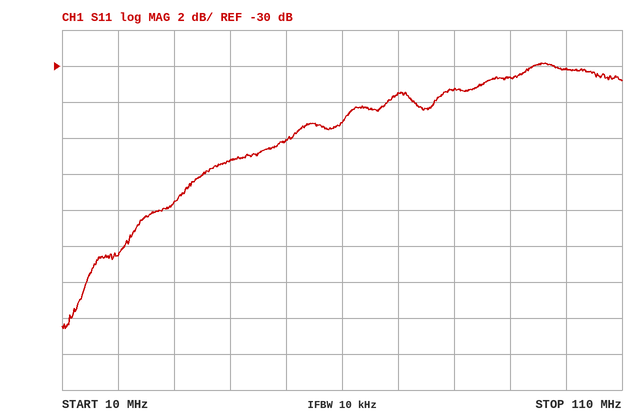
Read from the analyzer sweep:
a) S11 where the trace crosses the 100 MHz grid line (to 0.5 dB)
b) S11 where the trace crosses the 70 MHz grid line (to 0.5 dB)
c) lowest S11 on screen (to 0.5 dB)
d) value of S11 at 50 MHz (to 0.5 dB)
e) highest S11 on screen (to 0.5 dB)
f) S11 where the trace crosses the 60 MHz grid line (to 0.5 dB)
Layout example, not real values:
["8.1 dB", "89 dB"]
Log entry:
["-30.0 dB", "-31.5 dB", "-44.5 dB", "-34.0 dB", "-30.0 dB", "-33.0 dB"]
